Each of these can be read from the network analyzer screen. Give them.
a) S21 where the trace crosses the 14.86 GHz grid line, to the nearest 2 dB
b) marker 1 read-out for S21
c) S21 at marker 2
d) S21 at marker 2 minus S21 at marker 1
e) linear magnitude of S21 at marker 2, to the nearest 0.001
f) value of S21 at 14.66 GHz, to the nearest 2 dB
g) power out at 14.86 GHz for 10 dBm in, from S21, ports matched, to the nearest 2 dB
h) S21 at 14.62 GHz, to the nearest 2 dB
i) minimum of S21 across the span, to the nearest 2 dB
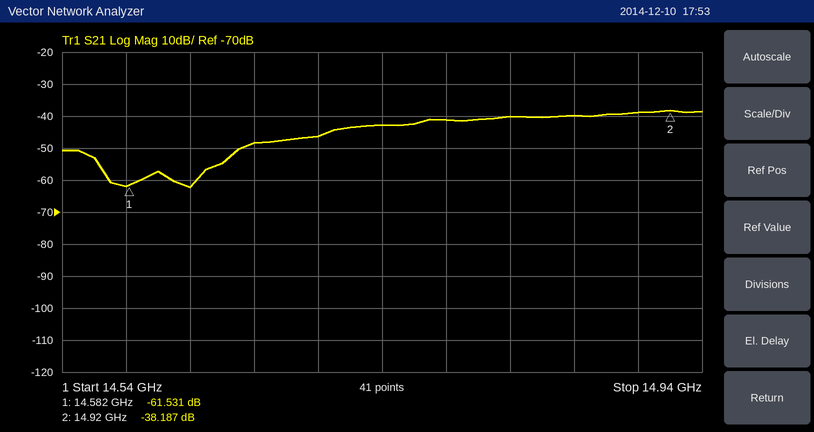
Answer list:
-40 dB
-61.531 dB
-38.187 dB
23.344 dB
0.012
-48 dB
-30 dBm
-62 dB
-62 dB
